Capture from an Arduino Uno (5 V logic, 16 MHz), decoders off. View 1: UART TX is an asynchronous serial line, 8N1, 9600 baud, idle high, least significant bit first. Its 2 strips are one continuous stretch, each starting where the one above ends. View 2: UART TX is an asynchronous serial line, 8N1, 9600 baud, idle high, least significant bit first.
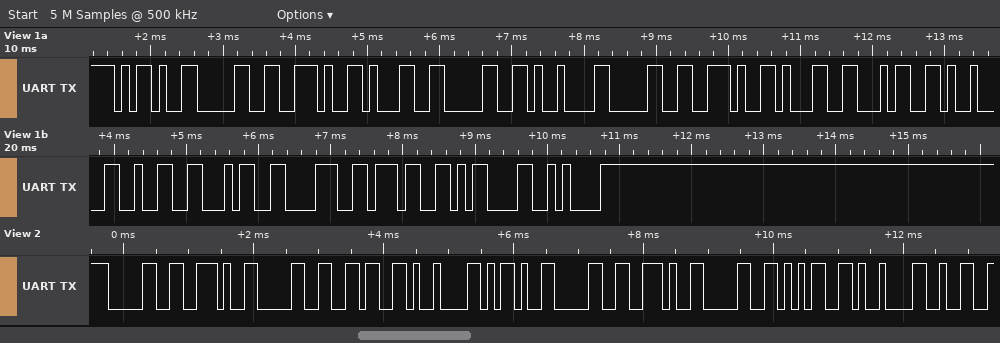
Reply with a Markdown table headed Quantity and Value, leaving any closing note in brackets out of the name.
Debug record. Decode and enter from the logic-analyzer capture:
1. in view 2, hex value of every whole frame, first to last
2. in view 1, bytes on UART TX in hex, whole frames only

| Quantity | Value |
|---|---|
| in view 2, hex value of every whole frame, first to last | 30 2E 30 36 09 2D 30 2E 30 35 09 32 |
| in view 1, bytes on UART TX in hex, whole frames only | 2D 30 2E 31 30 09 30 2E 31 34 09 32 34 38 37 0D 0A |
